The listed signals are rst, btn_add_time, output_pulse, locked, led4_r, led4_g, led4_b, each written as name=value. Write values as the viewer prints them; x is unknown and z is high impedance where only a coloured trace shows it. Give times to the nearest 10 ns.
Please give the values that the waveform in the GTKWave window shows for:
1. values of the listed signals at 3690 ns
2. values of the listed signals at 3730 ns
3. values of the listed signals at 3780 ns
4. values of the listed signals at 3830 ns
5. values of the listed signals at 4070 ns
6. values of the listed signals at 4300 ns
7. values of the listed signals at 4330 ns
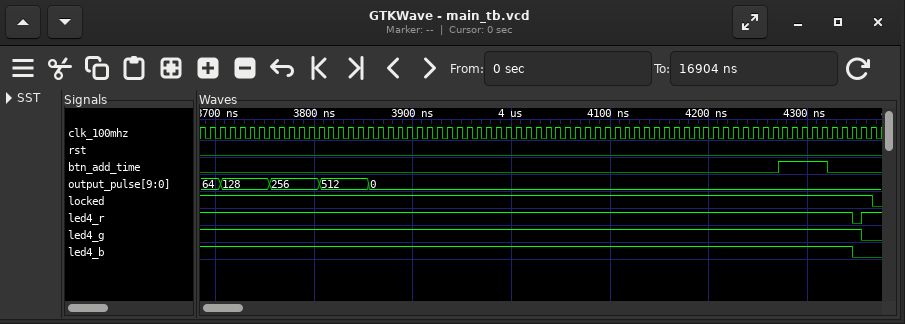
rst=0, btn_add_time=0, output_pulse=64, locked=1, led4_r=1, led4_g=1, led4_b=1
rst=0, btn_add_time=0, output_pulse=128, locked=1, led4_r=1, led4_g=1, led4_b=1
rst=0, btn_add_time=0, output_pulse=256, locked=1, led4_r=1, led4_g=1, led4_b=1
rst=0, btn_add_time=0, output_pulse=512, locked=1, led4_r=1, led4_g=1, led4_b=1
rst=0, btn_add_time=0, output_pulse=0, locked=1, led4_r=1, led4_g=1, led4_b=1
rst=0, btn_add_time=1, output_pulse=0, locked=1, led4_r=1, led4_g=1, led4_b=1
rst=0, btn_add_time=0, output_pulse=0, locked=1, led4_r=1, led4_g=1, led4_b=1
